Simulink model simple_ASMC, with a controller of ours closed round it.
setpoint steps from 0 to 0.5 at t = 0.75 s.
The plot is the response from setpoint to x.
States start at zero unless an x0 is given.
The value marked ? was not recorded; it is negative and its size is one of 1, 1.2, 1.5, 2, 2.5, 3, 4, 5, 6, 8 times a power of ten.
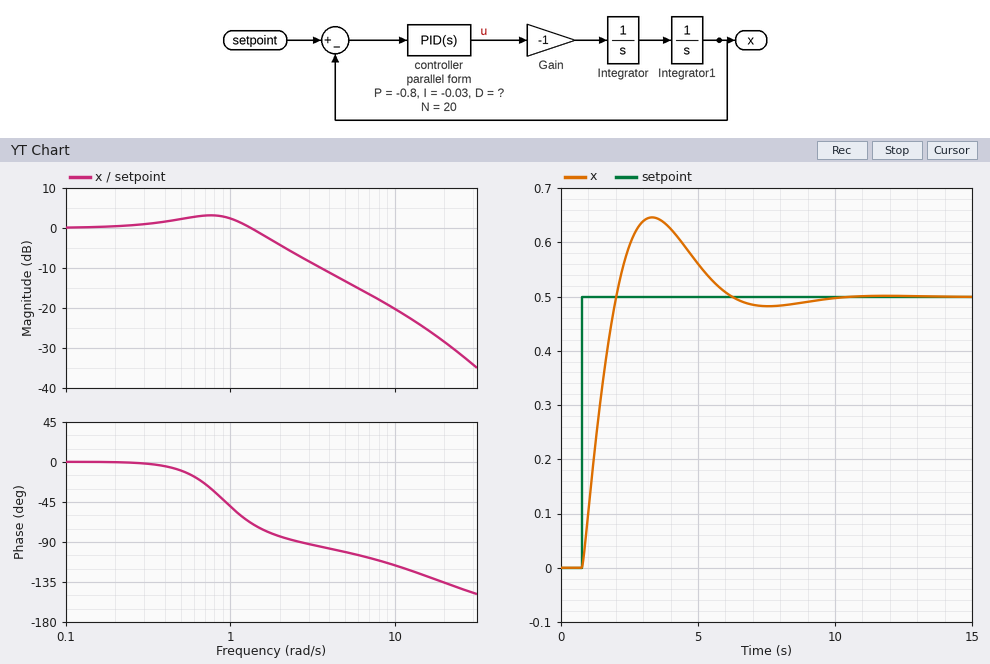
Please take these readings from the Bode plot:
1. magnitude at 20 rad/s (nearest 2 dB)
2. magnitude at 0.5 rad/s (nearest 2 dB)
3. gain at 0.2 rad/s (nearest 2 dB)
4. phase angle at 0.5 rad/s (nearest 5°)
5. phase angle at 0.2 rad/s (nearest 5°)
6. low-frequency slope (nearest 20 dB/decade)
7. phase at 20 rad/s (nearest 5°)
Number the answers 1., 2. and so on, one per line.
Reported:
1. -28 dB
2. 2 dB
3. 0 dB
4. -10°
5. 0°
6. 0 dB/decade
7. -135°
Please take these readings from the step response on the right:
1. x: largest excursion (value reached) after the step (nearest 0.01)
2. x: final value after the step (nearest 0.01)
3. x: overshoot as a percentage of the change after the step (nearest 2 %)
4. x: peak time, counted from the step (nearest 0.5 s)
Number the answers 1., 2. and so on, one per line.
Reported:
1. 0.65
2. 0.50
3. 30 %
4. 2.5 s
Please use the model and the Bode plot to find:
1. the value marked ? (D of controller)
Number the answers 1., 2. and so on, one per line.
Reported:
1. -1
